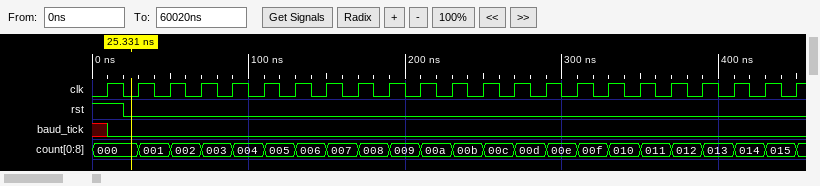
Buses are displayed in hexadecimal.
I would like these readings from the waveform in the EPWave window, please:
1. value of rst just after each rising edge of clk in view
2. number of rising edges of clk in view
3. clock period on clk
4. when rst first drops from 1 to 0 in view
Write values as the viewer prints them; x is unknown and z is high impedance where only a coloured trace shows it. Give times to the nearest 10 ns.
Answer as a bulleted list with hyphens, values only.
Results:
- 1 0 0 0 0 0 0 0 0 0 0 0 0 0 0 0 0 0 0 0 0 0 0
- 23
- 20 ns
- 20 ns
